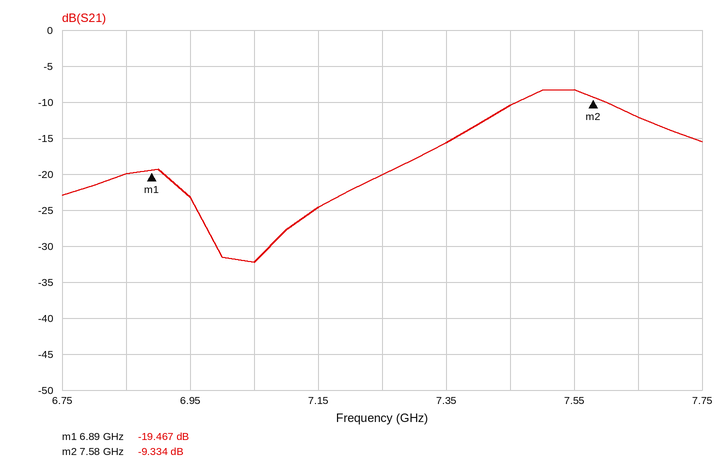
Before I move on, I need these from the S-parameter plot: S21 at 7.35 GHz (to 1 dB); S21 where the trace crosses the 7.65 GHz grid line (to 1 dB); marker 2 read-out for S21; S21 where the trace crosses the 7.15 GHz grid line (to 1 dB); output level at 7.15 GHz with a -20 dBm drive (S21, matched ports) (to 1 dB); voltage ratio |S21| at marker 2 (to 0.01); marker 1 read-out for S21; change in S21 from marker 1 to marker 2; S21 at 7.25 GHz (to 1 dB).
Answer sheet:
-16 dB
-12 dB
-9.334 dB
-25 dB
-45 dBm
0.34
-19.467 dB
10.133 dB
-20 dB
